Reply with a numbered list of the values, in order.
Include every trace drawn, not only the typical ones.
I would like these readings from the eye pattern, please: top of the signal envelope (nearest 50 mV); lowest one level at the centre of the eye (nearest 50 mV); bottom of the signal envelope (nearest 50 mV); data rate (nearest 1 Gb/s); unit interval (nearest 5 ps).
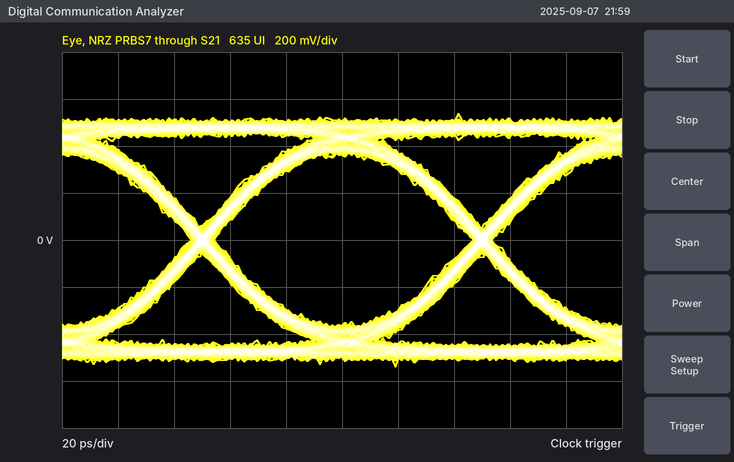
1. 550 mV
2. 350 mV
3. -550 mV
4. 10 Gb/s
5. 100 ps
